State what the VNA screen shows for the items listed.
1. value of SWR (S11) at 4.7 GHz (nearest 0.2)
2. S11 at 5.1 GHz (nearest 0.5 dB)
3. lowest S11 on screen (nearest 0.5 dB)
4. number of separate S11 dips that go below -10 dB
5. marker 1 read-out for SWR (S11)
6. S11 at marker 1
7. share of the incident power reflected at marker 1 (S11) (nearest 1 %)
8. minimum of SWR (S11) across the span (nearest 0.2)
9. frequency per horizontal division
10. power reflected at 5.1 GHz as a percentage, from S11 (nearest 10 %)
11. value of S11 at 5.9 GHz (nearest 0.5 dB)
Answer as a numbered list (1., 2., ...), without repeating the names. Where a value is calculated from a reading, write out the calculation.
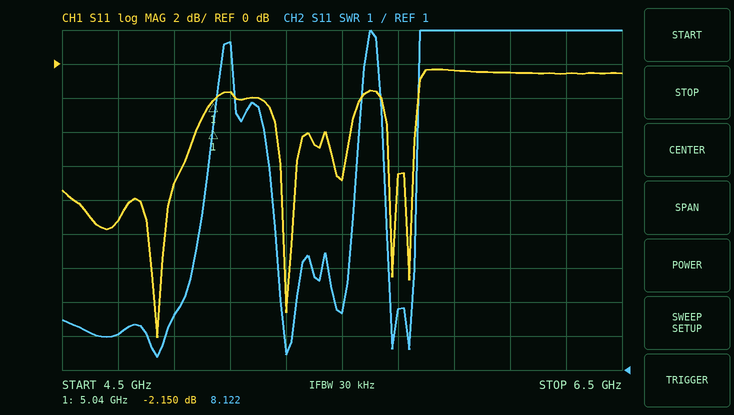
1. 2.0
2. -1.5 dB
3. -16.0 dB
4. 4
5. 8.122
6. -2.150 dB
7. 10^(-2.15/10) ≈ 61 %
8. 1.4
9. 200 MHz
10. 10^(-1.5/10) ≈ 70.8 %, so 70 % to the nearest 10 %
11. -0.5 dB
